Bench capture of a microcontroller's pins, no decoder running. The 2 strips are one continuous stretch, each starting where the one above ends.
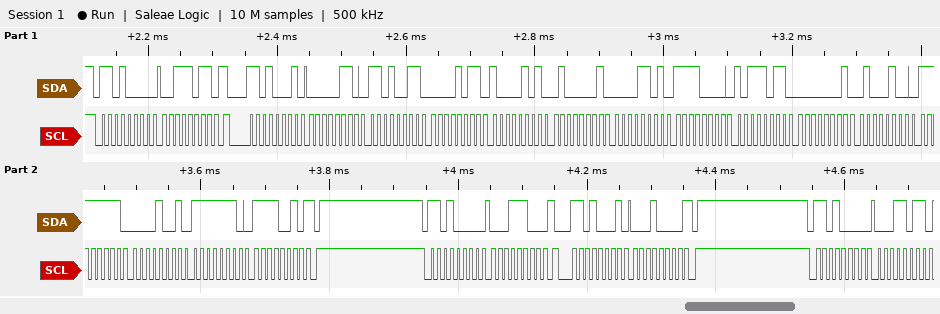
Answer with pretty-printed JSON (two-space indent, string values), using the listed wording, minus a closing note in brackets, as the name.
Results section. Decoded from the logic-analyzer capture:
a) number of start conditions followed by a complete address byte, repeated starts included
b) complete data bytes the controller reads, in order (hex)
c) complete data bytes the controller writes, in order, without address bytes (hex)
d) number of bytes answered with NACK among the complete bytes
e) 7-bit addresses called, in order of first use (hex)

{
  "number of start conditions followed by a complete address byte, repeated starts included": "5",
  "complete data bytes the controller reads, in order": "06 D3 0B 85 41 0D F0 BB 01 44 FF 09 FE F2 10",
  "complete data bytes the controller writes, in order, without address bytes": "3B 1C 1B",
  "number of bytes answered with NACK among the complete bytes": "2",
  "7-bit addresses called, in order of first use": "0x68"
}
